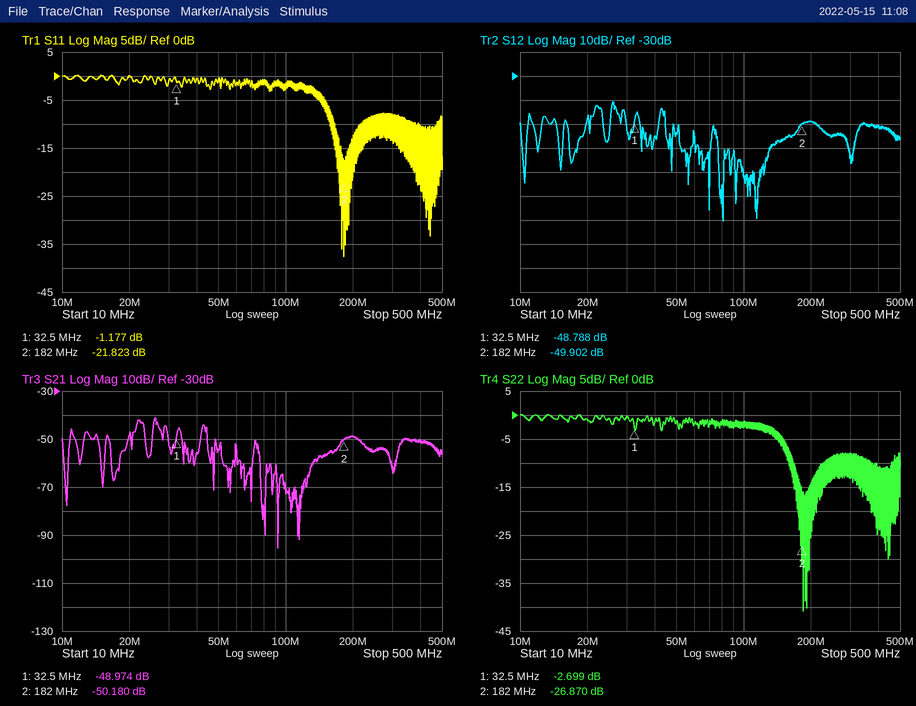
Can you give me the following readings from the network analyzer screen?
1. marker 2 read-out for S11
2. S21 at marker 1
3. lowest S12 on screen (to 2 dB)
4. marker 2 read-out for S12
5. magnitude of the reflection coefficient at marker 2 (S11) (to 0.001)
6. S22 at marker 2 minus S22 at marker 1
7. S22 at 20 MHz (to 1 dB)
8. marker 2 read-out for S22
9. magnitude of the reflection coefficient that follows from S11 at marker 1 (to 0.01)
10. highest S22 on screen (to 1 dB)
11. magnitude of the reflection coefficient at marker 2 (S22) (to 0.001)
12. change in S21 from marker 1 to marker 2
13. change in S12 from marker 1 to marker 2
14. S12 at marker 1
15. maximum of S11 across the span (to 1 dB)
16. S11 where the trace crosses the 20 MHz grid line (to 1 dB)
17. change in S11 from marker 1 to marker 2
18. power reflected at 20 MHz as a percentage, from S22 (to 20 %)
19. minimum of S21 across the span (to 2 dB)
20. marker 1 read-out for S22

-21.823 dB
-48.974 dB
-90 dB
-49.902 dB
0.081
-24.171 dB
-1 dB
-26.870 dB
0.87
0 dB
0.045
-1.206 dB
-1.114 dB
-48.788 dB
0 dB
0 dB
-20.646 dB
80 %
-96 dB
-2.699 dB
